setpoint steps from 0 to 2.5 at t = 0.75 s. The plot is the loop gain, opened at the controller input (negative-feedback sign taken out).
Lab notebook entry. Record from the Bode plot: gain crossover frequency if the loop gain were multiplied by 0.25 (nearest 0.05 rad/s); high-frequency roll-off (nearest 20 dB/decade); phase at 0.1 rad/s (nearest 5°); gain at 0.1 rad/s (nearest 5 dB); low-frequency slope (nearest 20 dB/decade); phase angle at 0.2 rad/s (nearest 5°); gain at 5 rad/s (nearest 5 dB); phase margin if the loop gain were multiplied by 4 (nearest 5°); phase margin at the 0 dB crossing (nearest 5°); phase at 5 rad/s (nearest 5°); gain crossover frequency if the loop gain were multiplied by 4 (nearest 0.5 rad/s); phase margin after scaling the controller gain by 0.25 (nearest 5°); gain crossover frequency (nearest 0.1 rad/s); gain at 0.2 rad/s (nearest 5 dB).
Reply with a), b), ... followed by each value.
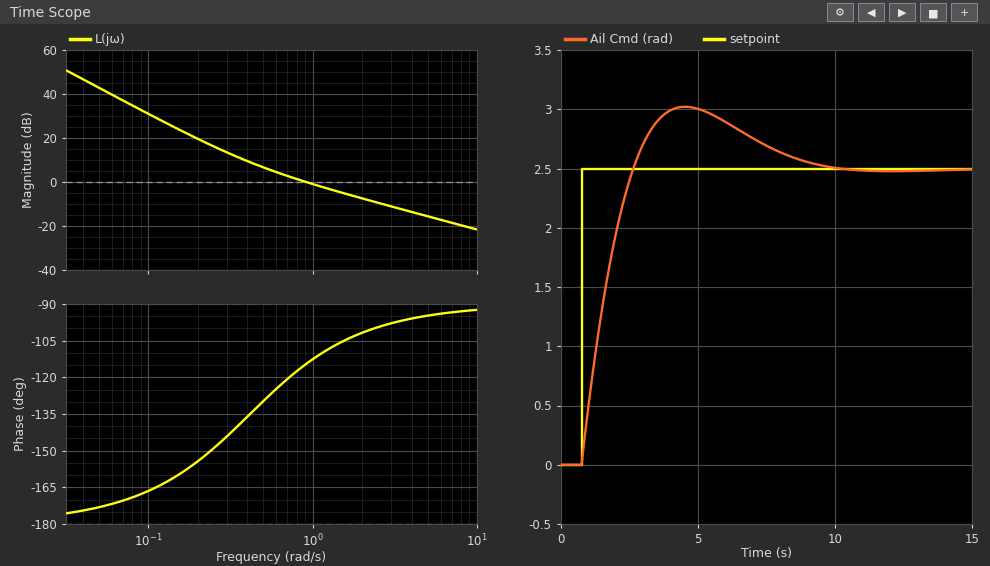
a) 0.35 rad/s
b) -20 dB/decade
c) -165°
d) 30 dB
e) -40 dB/decade
f) -155°
g) -15 dB
h) 85°
i) 65°
j) -95°
k) 3.5 rad/s
l) 40°
m) 0.9 rad/s
n) 20 dB
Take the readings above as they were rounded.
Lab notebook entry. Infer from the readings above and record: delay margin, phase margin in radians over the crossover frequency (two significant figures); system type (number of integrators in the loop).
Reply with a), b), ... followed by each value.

a) 1.3 s
b) 2
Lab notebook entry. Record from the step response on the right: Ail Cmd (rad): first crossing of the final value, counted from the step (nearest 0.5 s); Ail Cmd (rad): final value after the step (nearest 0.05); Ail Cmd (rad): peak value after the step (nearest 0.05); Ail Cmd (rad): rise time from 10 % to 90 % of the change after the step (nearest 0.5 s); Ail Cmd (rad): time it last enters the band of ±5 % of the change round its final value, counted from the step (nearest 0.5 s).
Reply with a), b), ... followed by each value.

a) 2.0 s
b) 2.50
c) 3.00
d) 1.5 s
e) 7.5 s
